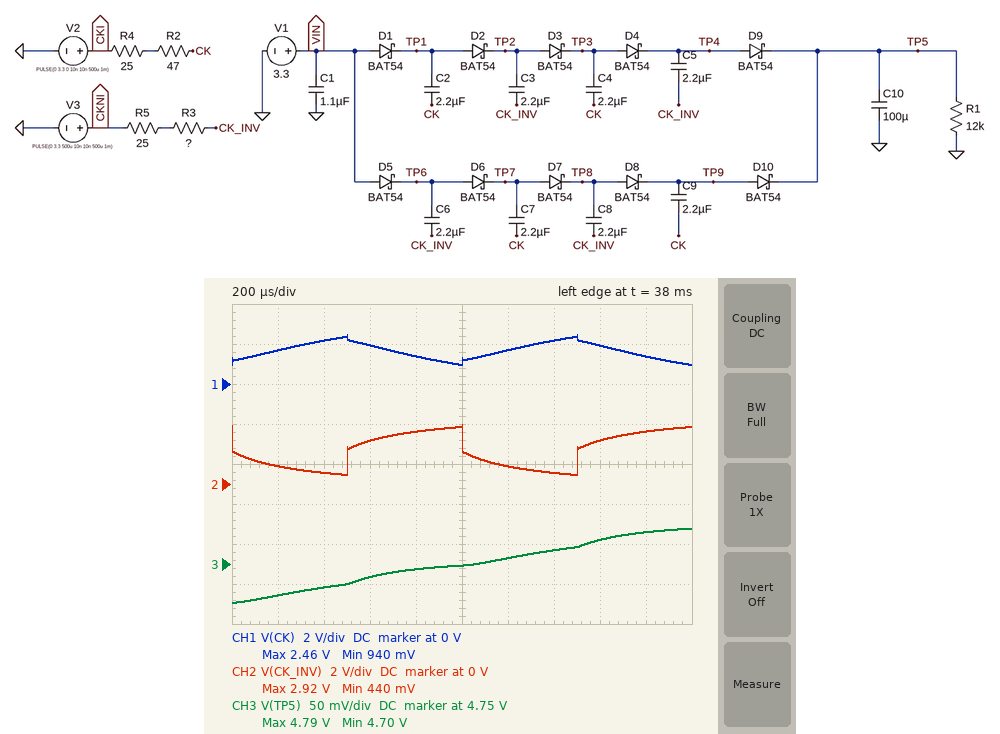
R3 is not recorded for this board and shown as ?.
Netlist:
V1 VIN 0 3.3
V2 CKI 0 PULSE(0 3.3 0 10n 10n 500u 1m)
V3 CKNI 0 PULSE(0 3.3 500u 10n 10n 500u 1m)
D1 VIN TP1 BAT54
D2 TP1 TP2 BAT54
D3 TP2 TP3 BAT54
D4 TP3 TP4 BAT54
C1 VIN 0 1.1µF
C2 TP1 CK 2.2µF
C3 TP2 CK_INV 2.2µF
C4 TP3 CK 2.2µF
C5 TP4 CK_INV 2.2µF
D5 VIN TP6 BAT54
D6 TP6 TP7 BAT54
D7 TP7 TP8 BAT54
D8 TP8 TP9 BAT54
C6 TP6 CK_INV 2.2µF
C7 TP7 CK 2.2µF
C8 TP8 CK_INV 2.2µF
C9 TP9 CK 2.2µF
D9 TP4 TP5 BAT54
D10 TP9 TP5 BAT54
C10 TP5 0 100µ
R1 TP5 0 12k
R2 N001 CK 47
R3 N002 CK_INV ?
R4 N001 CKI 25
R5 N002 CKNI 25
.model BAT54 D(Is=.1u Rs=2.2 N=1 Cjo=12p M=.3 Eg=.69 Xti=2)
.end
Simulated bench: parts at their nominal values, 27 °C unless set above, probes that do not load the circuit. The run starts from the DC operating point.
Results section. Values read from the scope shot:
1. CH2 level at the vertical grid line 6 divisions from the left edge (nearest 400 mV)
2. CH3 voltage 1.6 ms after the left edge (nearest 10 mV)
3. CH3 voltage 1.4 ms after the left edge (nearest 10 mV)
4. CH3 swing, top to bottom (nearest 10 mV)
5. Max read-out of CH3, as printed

800 mV
4.78 V
4.77 V
90 mV
4.79 V
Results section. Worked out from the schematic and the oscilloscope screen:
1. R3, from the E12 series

15 Ω
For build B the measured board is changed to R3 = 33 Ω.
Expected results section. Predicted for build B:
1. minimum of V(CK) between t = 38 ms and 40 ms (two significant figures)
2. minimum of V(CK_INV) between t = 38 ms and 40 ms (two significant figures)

900 mV
690 mV
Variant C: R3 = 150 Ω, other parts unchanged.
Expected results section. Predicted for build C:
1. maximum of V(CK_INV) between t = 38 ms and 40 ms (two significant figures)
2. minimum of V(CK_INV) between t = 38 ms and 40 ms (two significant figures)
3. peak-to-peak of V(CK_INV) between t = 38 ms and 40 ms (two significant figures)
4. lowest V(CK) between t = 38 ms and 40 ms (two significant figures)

2.0 V
1.3 V
670 mV
660 mV
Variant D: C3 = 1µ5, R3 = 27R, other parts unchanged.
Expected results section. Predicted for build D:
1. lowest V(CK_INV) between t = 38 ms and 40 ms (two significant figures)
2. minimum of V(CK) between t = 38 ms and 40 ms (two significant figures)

590 mV
890 mV
